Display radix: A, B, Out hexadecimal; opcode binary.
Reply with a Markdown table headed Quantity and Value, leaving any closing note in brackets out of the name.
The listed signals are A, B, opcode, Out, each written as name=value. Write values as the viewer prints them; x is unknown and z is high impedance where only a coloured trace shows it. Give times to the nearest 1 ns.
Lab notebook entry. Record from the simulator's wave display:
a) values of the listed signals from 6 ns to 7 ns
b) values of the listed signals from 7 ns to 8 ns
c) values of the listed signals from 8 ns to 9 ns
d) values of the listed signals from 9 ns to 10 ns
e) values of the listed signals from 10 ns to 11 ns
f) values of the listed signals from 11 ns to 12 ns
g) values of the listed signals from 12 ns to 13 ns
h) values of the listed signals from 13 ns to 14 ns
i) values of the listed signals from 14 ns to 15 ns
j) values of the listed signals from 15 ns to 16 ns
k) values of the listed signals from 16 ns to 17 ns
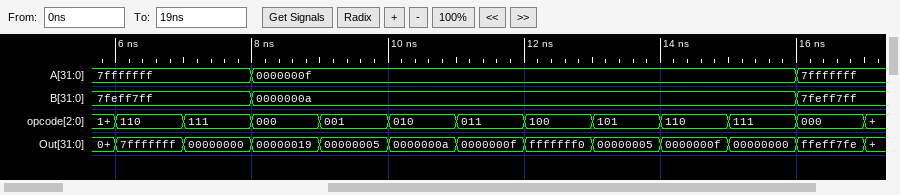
| Quantity | Value |
|---|---|
| values of the listed signals from 6 ns to 7 ns | A=7fffffff, B=7feff7ff, opcode=110, Out=7fffffff |
| values of the listed signals from 7 ns to 8 ns | A=7fffffff, B=7feff7ff, opcode=111, Out=00000000 |
| values of the listed signals from 8 ns to 9 ns | A=0000000f, B=0000000a, opcode=000, Out=00000019 |
| values of the listed signals from 9 ns to 10 ns | A=0000000f, B=0000000a, opcode=001, Out=00000005 |
| values of the listed signals from 10 ns to 11 ns | A=0000000f, B=0000000a, opcode=010, Out=0000000a |
| values of the listed signals from 11 ns to 12 ns | A=0000000f, B=0000000a, opcode=011, Out=0000000f |
| values of the listed signals from 12 ns to 13 ns | A=0000000f, B=0000000a, opcode=100, Out=fffffff0 |
| values of the listed signals from 13 ns to 14 ns | A=0000000f, B=0000000a, opcode=101, Out=00000005 |
| values of the listed signals from 14 ns to 15 ns | A=0000000f, B=0000000a, opcode=110, Out=0000000f |
| values of the listed signals from 15 ns to 16 ns | A=0000000f, B=0000000a, opcode=111, Out=00000000 |
| values of the listed signals from 16 ns to 17 ns | A=7fffffff, B=7feff7ff, opcode=000, Out=ffeff7fe |
